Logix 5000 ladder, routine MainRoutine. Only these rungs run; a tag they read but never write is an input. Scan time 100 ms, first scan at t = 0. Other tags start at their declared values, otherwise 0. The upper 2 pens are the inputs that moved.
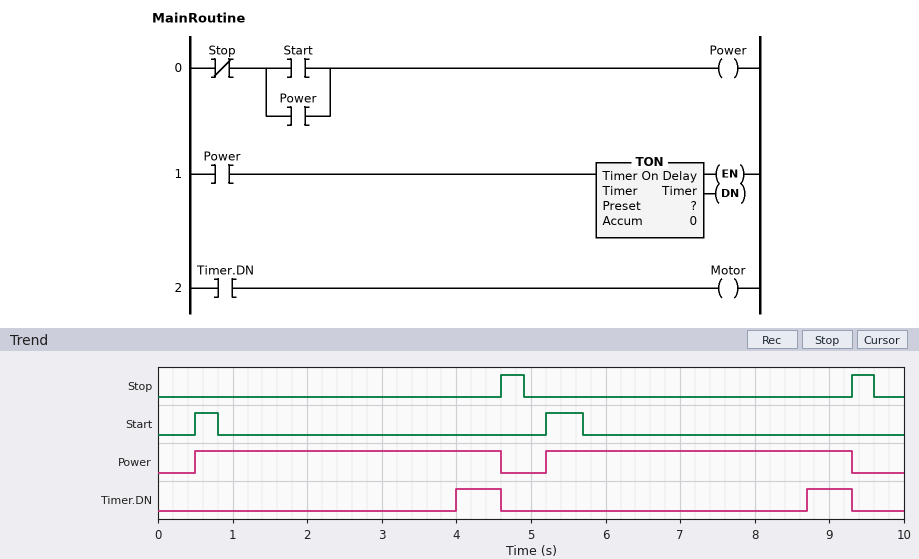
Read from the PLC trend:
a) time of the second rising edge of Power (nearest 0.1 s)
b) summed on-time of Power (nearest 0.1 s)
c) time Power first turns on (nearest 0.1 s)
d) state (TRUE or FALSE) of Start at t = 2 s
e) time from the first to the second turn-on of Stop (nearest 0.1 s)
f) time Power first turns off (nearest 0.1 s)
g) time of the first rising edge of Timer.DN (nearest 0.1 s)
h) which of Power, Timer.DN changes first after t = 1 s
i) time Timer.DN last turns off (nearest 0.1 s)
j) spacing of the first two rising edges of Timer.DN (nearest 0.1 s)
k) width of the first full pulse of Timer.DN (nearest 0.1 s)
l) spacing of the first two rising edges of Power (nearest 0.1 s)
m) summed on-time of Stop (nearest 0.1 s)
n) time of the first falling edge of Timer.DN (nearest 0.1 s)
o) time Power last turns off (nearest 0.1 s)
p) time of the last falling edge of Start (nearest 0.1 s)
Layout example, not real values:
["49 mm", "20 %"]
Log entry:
["5.2 s", "8.2 s", "0.5 s", "FALSE", "4.7 s", "4.6 s", "4.0 s", "Timer.DN", "9.3 s", "4.7 s", "0.6 s", "4.7 s", "0.6 s", "4.6 s", "9.3 s", "5.7 s"]
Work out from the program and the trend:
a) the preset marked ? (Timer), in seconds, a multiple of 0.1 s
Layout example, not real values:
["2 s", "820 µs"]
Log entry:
["3.5 s"]
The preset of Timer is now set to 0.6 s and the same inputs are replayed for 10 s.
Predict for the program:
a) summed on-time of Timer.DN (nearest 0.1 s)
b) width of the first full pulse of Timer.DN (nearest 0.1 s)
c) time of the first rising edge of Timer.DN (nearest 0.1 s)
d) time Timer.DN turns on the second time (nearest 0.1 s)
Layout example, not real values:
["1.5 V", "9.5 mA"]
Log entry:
["7.0 s", "3.5 s", "1.1 s", "5.8 s"]
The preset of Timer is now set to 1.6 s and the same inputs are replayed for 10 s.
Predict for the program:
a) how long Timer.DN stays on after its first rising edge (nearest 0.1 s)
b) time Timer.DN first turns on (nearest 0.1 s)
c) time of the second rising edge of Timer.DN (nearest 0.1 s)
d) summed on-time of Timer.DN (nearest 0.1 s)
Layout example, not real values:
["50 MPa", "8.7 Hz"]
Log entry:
["2.5 s", "2.1 s", "6.8 s", "5.0 s"]
